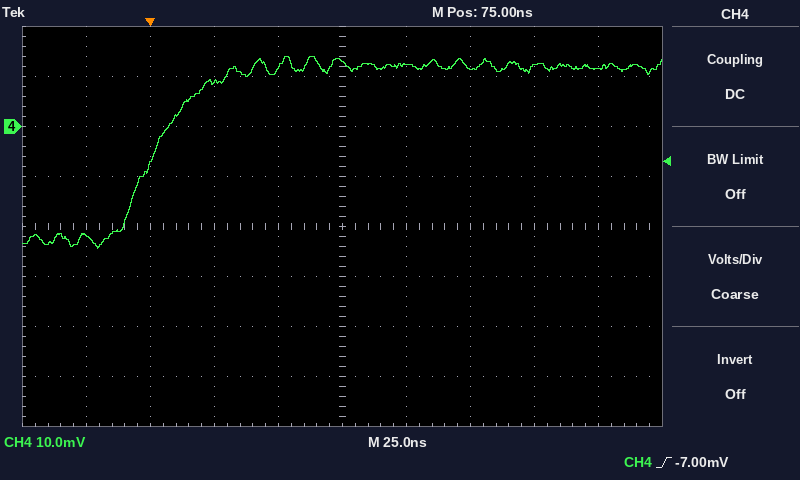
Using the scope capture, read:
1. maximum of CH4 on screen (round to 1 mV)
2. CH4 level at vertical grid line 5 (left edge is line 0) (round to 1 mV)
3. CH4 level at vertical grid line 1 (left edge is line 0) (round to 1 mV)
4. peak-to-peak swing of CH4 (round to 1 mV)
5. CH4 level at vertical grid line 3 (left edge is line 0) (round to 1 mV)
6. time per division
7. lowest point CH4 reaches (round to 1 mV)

14 mV
13 mV
-22 mV
38 mV
9 mV
25 ns
-24 mV
